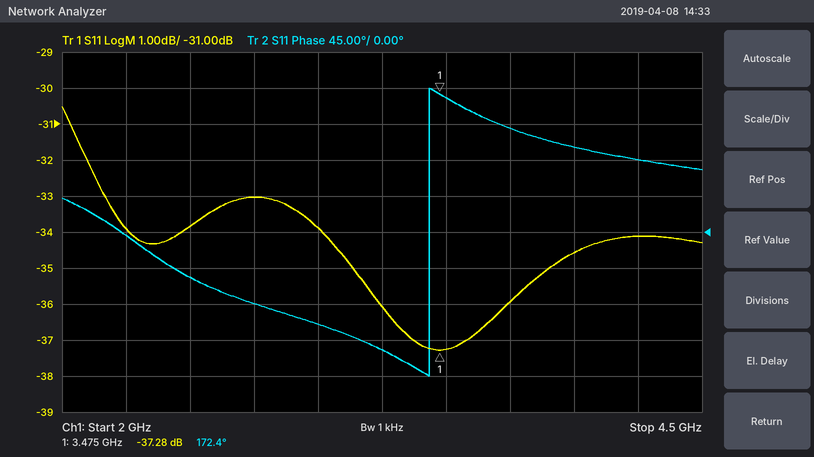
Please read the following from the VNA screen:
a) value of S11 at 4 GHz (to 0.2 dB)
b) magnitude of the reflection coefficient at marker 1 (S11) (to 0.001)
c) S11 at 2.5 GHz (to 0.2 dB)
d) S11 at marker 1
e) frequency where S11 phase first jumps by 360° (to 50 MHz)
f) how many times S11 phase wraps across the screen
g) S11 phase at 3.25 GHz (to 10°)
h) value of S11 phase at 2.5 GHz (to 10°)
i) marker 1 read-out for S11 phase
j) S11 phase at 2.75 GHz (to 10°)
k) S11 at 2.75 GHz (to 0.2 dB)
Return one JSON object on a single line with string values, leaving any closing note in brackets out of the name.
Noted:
{"value of S11 at 4 GHz": "-34.6 dB", "magnitude of the reflection coefficient at marker 1 (S11)": "0.014", "S11 at 2.5 GHz": "-33.8 dB", "S11 at marker 1": "-37.28 dB", "frequency where S11 phase first jumps by 360°": "3.45 GHz", "how many times S11 phase wraps across the screen": "1", "S11 phase at 3.25 GHz": "-150°", "value of S11 phase at 2.5 GHz": "-60°", "marker 1 read-out for S11 phase": "172.4°", "S11 phase at 2.75 GHz": "-90°", "S11 at 2.75 GHz": "-33.0 dB"}
